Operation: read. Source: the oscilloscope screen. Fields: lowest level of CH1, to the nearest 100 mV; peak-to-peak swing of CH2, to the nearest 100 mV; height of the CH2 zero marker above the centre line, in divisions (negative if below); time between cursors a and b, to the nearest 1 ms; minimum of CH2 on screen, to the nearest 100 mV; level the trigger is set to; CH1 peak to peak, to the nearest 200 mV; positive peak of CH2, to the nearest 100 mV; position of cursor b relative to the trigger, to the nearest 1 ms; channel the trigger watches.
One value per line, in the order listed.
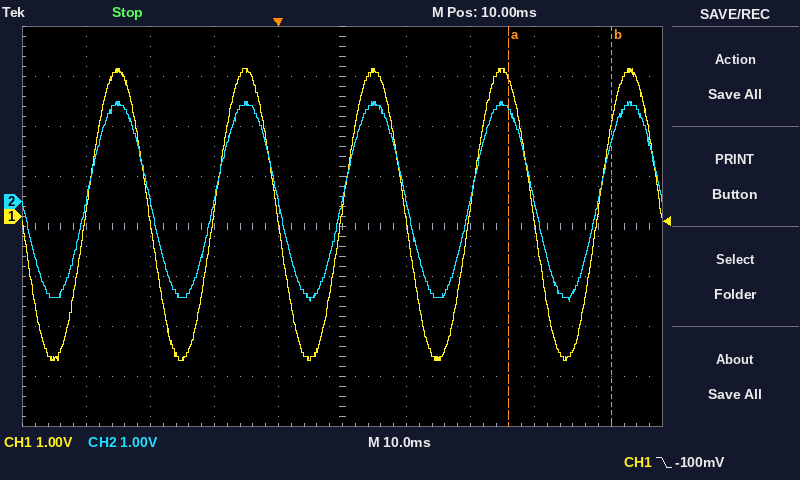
-2.9 V
4.0 V
+0.5 div
16 ms
-2.0 V
-100 mV
5.8 V
2.0 V
+52 ms
CH1
